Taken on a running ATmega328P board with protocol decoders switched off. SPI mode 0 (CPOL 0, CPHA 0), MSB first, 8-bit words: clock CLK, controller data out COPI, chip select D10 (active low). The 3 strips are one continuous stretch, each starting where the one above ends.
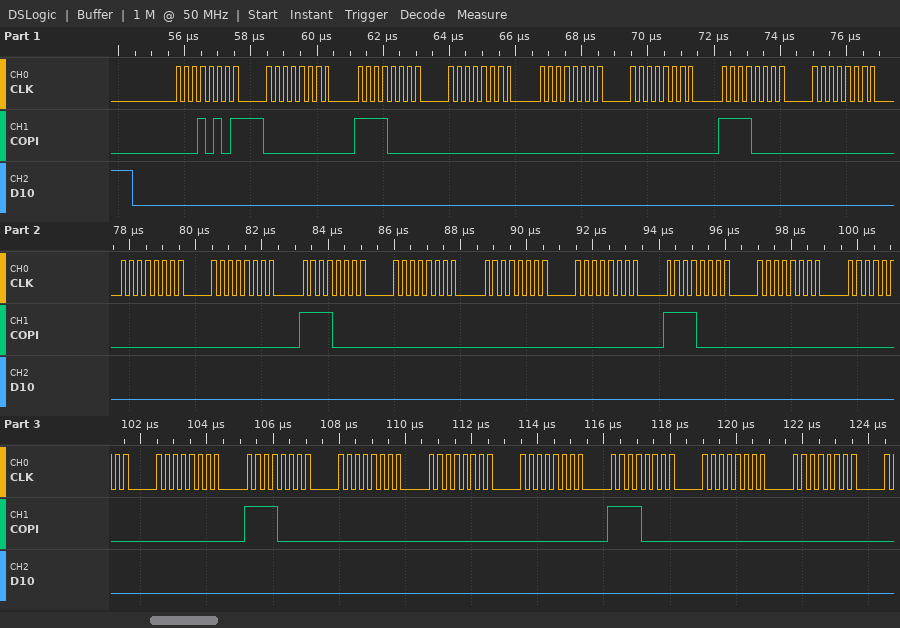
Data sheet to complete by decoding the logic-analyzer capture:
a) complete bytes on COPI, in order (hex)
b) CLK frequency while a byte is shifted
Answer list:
15 00 F0 00 00 00 F0 00 00 00 F0 00 00 00 F0 00 00 00 F0 00 00 00 F0 00 00
4 MHz
